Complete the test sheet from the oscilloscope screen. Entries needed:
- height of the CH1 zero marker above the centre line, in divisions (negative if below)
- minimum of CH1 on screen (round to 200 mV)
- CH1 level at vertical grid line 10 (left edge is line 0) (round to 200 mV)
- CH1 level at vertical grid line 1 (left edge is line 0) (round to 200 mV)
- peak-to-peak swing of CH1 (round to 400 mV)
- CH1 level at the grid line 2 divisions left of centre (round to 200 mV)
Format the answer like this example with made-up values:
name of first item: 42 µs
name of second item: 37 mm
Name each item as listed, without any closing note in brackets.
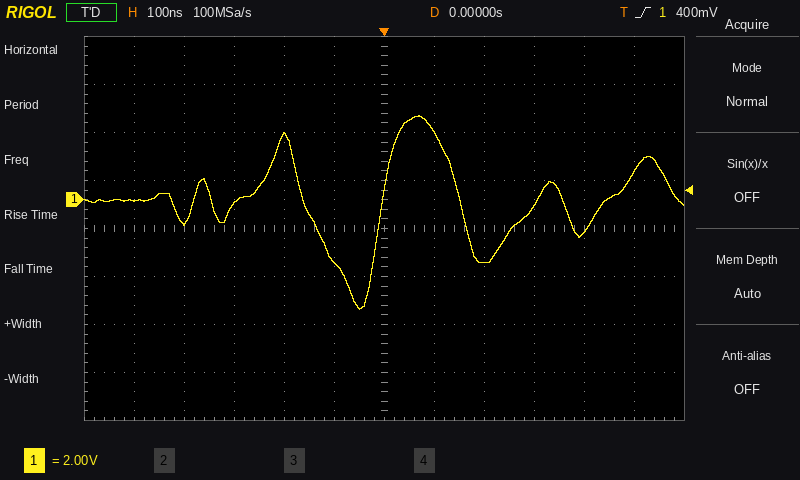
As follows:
height of the CH1 zero marker above the centre line, in divisions: +0.6 div
minimum of CH1 on screen: -4.6 V
CH1 level at vertical grid line 10 (left edge is line 0): -1.4 V
CH1 level at vertical grid line 1 (left edge is line 0): 0.0 V
peak-to-peak swing of CH1: 8.0 V
CH1 level at the grid line 2 divisions left of centre: 2.6 V
